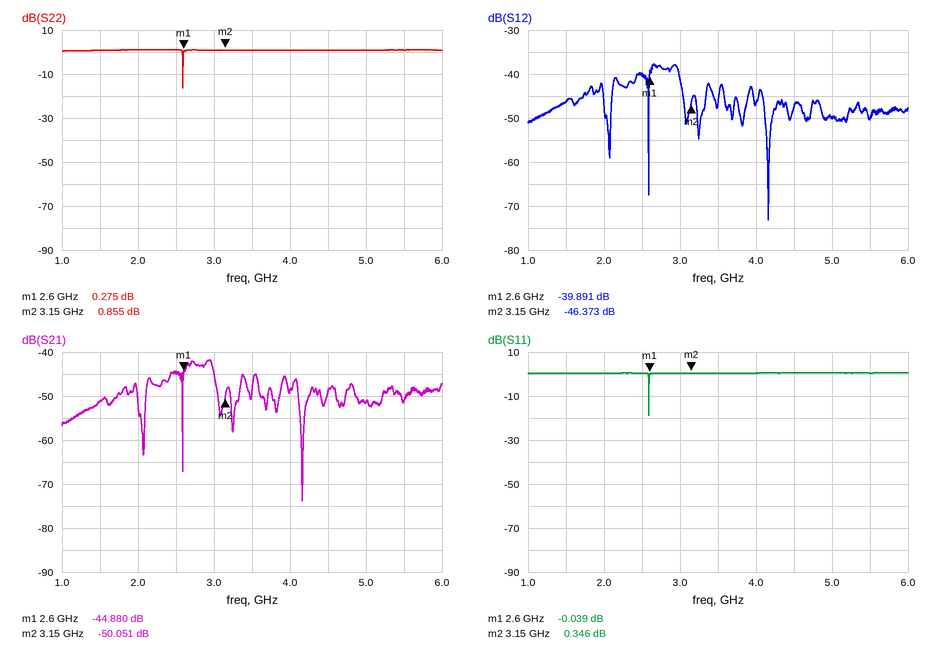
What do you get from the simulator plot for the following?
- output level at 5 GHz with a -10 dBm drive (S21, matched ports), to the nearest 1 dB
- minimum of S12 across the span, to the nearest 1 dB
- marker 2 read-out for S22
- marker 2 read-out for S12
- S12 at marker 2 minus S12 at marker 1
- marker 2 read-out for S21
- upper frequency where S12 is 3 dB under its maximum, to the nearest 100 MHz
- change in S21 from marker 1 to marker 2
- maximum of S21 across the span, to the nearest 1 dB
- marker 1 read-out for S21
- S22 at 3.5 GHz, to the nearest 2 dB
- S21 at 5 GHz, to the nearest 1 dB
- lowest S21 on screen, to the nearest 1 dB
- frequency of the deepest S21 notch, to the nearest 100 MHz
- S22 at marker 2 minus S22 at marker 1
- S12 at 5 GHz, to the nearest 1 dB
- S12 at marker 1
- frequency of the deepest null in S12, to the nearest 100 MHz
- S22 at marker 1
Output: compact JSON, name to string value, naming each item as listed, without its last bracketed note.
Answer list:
{"output level at 5 GHz with a -10 dBm drive (S21, matched ports), to the nearest 1 dB": "-61 dBm", "minimum of S12 across the span, to the nearest 1 dB": "-73 dB", "marker 2 read-out for S22": "0.855 dB", "marker 2 read-out for S12": "-46.373 dB", "S12 at marker 2 minus S12 at marker 1": "-6.482 dB", "marker 2 read-out for S21": "-50.051 dB", "upper frequency where S12 is 3 dB under its maximum, to the nearest 100 MHz": "3.0 GHz", "change in S21 from marker 1 to marker 2": "-5.171 dB", "maximum of S21 across the span, to the nearest 1 dB": "-42 dB", "marker 1 read-out for S21": "-44.880 dB", "S22 at 3.5 GHz, to the nearest 2 dB": "0 dB", "S21 at 5 GHz, to the nearest 1 dB": "-51 dB", "lowest S21 on screen, to the nearest 1 dB": "-74 dB", "frequency of the deepest S21 notch, to the nearest 100 MHz": "4.2 GHz", "S22 at marker 2 minus S22 at marker 1": "0.580 dB", "S12 at 5 GHz, to the nearest 1 dB": "-50 dB", "S12 at marker 1": "-39.891 dB", "frequency of the deepest null in S12, to the nearest 100 MHz": "4.2 GHz", "S22 at marker 1": "0.275 dB"}
